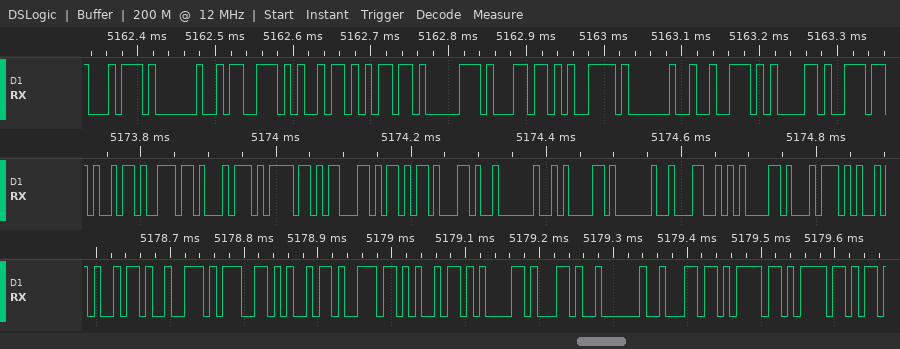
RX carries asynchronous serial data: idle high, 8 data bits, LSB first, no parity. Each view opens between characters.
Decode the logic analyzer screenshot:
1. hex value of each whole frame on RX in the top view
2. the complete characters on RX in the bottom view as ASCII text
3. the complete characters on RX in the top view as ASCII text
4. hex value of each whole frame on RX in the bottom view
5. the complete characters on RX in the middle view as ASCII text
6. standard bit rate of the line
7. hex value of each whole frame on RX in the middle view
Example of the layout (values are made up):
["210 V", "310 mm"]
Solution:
["74, 20, 73, 69, 6D, 70, 6C, 79, 20, 72, 61", "\"irginia, loo\"", "\"t simply ra\"", "69, 72, 67, 69, 6E, 69, 61, 2C, 20, 6C, 6F, 6F", "\"intock, a Lat\"", "115200 baud", "69, 6E, 74, 6F, 63, 6B, 2C, 20, 61, 20, 4C, 61, 74"]
